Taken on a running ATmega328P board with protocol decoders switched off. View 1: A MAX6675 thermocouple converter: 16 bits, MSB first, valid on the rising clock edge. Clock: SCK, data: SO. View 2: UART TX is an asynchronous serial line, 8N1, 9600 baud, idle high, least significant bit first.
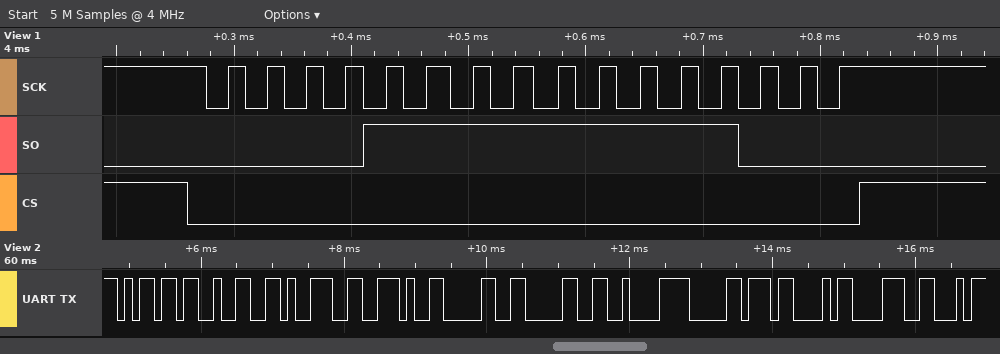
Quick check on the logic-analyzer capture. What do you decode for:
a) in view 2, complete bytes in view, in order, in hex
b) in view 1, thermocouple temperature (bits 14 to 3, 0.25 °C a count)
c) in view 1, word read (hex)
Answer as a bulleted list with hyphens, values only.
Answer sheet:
- 6D 32 39 2E 30 30 C2 B0 43 38
- 127.75 °C
- 0x0FF8
